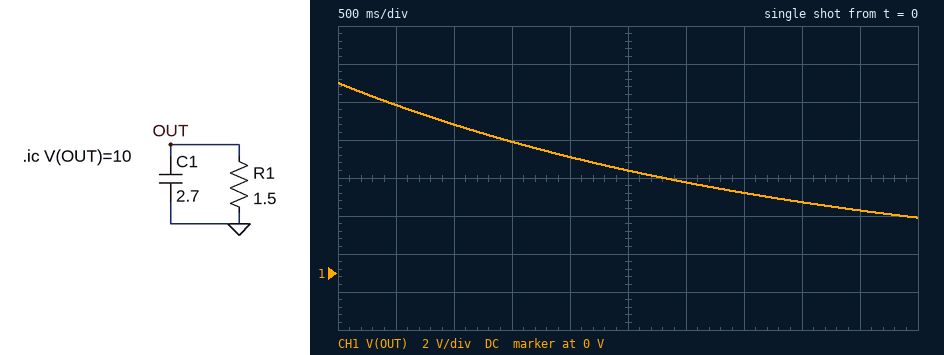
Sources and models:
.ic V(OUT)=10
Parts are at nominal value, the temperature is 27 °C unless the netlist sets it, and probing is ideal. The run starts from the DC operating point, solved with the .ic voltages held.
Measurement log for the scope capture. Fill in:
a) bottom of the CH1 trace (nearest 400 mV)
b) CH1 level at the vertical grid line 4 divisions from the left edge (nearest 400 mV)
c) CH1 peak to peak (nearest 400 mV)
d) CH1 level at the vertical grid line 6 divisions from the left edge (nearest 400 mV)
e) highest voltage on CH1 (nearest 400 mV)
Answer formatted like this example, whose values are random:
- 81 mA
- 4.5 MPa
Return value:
- 2.8 V
- 6.0 V
- 7.2 V
- 4.8 V
- 10.0 V
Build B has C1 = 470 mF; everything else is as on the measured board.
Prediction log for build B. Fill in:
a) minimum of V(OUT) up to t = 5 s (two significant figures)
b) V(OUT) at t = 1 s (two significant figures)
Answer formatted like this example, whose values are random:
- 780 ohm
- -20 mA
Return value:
- 8.3 mV
- 2.4 V
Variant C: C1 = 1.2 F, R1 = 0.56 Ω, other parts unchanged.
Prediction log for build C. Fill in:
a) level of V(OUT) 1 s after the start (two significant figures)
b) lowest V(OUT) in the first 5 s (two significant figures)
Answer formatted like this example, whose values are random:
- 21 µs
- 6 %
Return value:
- 2.3 V
- 5.9 mV
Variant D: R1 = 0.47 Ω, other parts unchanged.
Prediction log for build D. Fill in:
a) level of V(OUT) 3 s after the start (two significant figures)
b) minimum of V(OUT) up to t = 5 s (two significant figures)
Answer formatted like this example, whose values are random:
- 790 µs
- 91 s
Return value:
- 940 mV
- 190 mV
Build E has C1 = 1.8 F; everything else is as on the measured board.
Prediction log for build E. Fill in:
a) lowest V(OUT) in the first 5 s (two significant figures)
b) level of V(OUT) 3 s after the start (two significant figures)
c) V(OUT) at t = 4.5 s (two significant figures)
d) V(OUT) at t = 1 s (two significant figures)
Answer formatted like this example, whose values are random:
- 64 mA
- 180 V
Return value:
- 1.6 V
- 3.3 V
- 1.9 V
- 6.9 V
